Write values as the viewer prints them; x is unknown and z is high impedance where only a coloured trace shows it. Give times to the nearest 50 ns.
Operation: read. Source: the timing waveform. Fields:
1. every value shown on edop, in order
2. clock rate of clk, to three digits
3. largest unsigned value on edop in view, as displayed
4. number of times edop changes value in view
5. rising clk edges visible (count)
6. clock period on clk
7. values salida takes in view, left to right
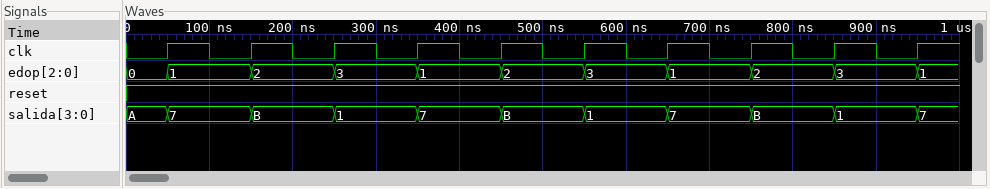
0, 1, 2, 3, 1, 2, 3, 1, 2, 3, 1
10.0 MHz
3
10
10
100 ns
A, 7, B, 1, 7, B, 1, 7, B, 1, 7
